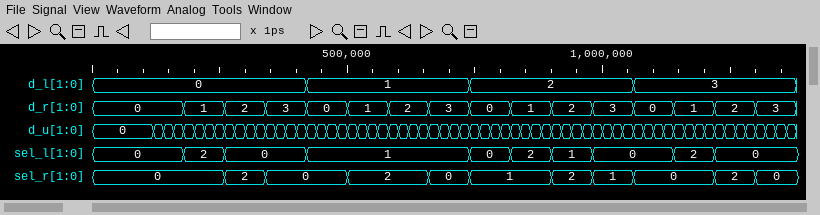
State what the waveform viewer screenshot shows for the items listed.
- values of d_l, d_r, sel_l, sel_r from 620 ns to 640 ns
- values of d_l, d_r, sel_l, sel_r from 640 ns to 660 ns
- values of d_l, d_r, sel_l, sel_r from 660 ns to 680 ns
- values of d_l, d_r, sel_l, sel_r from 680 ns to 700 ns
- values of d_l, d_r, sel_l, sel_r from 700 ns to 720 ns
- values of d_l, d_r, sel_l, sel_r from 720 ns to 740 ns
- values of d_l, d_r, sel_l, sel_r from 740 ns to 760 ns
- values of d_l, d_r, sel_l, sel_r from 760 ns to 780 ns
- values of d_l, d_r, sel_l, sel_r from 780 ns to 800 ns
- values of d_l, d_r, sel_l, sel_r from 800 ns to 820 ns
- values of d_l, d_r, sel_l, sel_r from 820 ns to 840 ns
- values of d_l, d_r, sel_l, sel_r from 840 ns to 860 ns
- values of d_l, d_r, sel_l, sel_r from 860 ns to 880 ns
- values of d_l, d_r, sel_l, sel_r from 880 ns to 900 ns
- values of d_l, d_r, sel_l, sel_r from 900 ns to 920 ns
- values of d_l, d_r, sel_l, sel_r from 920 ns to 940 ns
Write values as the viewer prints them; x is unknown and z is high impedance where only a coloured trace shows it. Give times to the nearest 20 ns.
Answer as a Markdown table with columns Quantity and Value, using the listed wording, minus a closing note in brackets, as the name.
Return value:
| Quantity | Value |
|---|---|
| values of d_l, d_r, sel_l, sel_r from 620 ns to 640 ns | d_l=1, d_r=2, sel_l=1, sel_r=2 |
| values of d_l, d_r, sel_l, sel_r from 640 ns to 660 ns | d_l=1, d_r=2, sel_l=1, sel_r=2 |
| values of d_l, d_r, sel_l, sel_r from 660 ns to 680 ns | d_l=1, d_r=3, sel_l=1, sel_r=0 |
| values of d_l, d_r, sel_l, sel_r from 680 ns to 700 ns | d_l=1, d_r=3, sel_l=1, sel_r=0 |
| values of d_l, d_r, sel_l, sel_r from 700 ns to 720 ns | d_l=1, d_r=3, sel_l=1, sel_r=0 |
| values of d_l, d_r, sel_l, sel_r from 720 ns to 740 ns | d_l=1, d_r=3, sel_l=1, sel_r=0 |
| values of d_l, d_r, sel_l, sel_r from 740 ns to 760 ns | d_l=2, d_r=0, sel_l=0, sel_r=1 |
| values of d_l, d_r, sel_l, sel_r from 760 ns to 780 ns | d_l=2, d_r=0, sel_l=0, sel_r=1 |
| values of d_l, d_r, sel_l, sel_r from 780 ns to 800 ns | d_l=2, d_r=0, sel_l=0, sel_r=1 |
| values of d_l, d_r, sel_l, sel_r from 800 ns to 820 ns | d_l=2, d_r=0, sel_l=0, sel_r=1 |
| values of d_l, d_r, sel_l, sel_r from 820 ns to 840 ns | d_l=2, d_r=1, sel_l=2, sel_r=1 |
| values of d_l, d_r, sel_l, sel_r from 840 ns to 860 ns | d_l=2, d_r=1, sel_l=2, sel_r=1 |
| values of d_l, d_r, sel_l, sel_r from 860 ns to 880 ns | d_l=2, d_r=1, sel_l=2, sel_r=1 |
| values of d_l, d_r, sel_l, sel_r from 880 ns to 900 ns | d_l=2, d_r=1, sel_l=2, sel_r=1 |
| values of d_l, d_r, sel_l, sel_r from 900 ns to 920 ns | d_l=2, d_r=2, sel_l=1, sel_r=2 |
| values of d_l, d_r, sel_l, sel_r from 920 ns to 940 ns | d_l=2, d_r=2, sel_l=1, sel_r=2 |
